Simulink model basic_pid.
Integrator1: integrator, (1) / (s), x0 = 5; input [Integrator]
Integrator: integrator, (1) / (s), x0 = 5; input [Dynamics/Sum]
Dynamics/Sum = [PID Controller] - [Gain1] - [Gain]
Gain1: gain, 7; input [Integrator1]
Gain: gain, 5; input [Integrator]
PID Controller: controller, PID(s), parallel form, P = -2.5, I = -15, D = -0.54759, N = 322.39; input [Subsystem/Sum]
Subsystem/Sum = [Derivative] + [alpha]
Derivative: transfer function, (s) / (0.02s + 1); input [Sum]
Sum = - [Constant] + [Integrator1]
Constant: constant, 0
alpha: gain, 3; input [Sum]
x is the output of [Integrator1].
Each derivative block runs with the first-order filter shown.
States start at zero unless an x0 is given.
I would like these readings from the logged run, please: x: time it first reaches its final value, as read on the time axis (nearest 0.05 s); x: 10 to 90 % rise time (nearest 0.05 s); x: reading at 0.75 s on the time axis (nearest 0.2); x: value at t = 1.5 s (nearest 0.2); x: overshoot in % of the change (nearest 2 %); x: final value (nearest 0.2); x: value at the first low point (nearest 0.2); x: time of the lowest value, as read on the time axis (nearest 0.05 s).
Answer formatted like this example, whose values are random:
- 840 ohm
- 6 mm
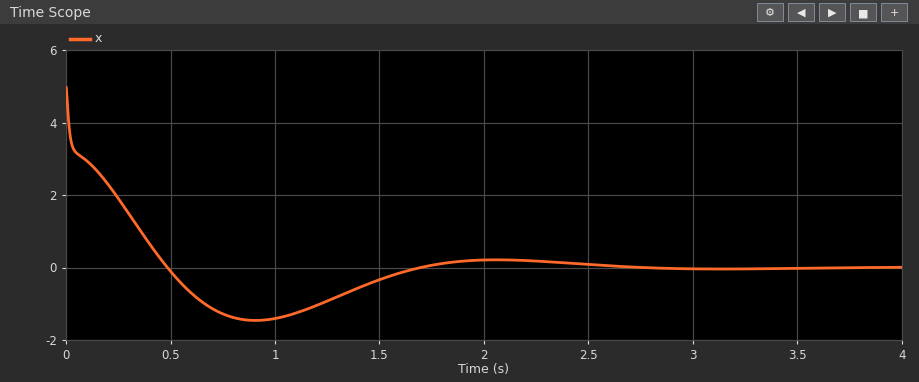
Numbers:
- 0.50 s
- 0.40 s
- -1.2
- -0.4
- 30 %
- 0.0
- -1.4
- 0.90 s
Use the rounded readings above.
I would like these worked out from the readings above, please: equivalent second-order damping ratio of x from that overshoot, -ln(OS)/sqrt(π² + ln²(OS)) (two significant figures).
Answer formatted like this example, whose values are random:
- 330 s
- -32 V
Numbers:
- 0.36
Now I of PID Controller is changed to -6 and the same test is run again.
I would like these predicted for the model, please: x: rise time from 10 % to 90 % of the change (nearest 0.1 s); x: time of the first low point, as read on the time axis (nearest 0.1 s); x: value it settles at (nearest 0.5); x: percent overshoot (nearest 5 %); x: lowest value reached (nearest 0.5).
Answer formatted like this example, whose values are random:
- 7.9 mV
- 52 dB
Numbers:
- 0.6 s
- 1.3 s
- 0.0
- 20 %
- -1.0
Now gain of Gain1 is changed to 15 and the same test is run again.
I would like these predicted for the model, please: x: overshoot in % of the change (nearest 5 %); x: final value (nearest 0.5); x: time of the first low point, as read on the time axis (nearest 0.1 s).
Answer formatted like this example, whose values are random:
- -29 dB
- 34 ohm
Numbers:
- 25 %
- 0.0
- 0.8 s
